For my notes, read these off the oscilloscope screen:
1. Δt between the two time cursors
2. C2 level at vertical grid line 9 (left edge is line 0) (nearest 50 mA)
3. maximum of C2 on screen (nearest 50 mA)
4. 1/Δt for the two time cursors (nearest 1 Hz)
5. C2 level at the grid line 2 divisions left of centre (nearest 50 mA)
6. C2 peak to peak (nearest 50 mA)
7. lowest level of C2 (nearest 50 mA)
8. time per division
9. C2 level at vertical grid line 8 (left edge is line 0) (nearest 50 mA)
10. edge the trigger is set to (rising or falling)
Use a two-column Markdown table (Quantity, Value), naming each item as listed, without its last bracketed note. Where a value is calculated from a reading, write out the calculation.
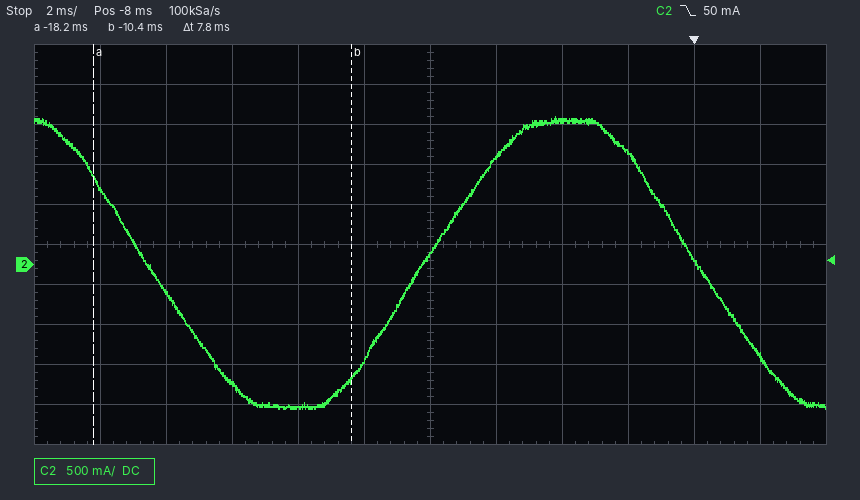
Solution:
| Quantity | Value |
|---|---|
| Δt between the two time cursors | 7.8 ms |
| C2 level at vertical grid line 9 (left edge is line 0) | 1.40 A |
| maximum of C2 on screen | 1.85 A |
| 1/Δt for the two time cursors | 1 / 7.8 ms ≈ 128 Hz |
| C2 level at the grid line 2 divisions left of centre | -1.80 A |
| C2 peak to peak | 1.85 A − (-1.80 A) = 3.65 A |
| lowest level of C2 | -1.80 A |
| time per division | 2 ms |
| C2 level at vertical grid line 8 (left edge is line 0) | 1.80 A |
| edge the trigger is set to | falling |
